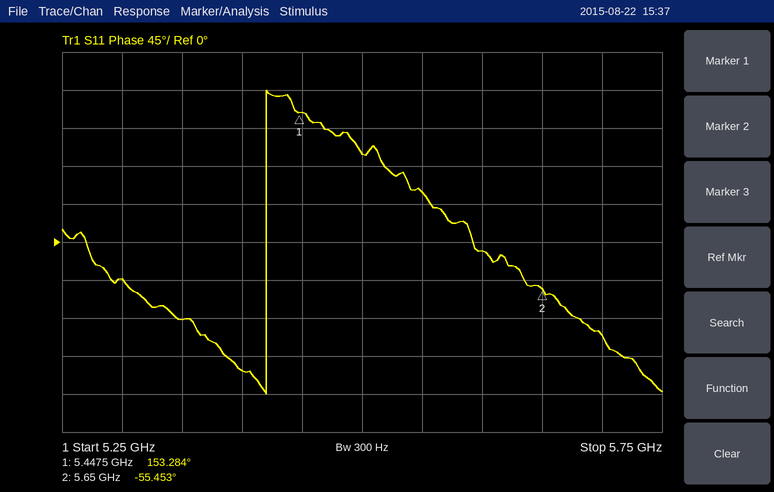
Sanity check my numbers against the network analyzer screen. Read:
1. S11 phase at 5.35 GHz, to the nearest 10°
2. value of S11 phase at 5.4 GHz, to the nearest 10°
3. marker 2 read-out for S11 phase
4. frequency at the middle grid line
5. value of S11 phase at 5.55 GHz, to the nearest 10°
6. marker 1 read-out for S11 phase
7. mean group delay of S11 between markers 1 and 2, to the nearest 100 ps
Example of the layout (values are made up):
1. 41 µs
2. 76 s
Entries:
1. -90°
2. -150°
3. -55.453°
4. 5.5 GHz
5. 60°
6. 153.284°
7. 2.9 ns
